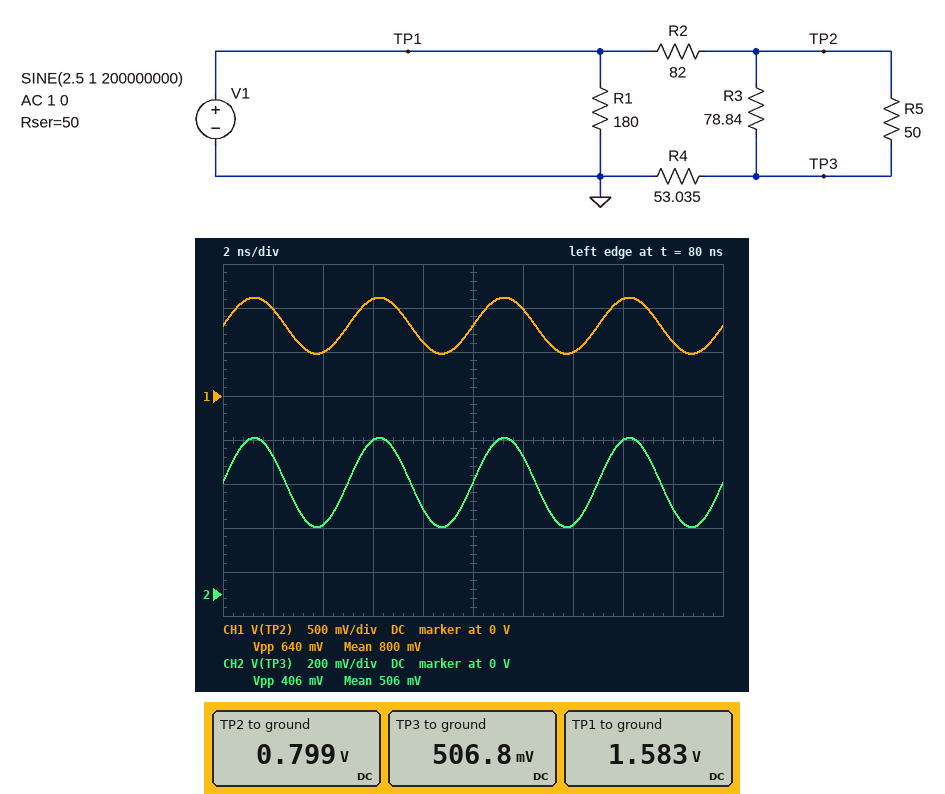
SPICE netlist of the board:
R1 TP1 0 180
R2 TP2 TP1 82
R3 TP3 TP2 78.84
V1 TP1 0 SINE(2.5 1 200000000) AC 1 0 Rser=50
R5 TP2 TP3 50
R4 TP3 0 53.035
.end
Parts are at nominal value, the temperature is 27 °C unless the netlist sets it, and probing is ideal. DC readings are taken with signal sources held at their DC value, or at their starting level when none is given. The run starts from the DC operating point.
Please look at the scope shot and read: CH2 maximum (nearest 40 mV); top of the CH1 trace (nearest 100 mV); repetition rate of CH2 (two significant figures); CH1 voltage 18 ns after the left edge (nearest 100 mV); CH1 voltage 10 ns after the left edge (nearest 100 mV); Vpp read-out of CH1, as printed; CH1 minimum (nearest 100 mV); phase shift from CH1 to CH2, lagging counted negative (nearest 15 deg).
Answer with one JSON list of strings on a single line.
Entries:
["720 mV", "1.1 V", "200 MHz", "600 mV", "800 mV", "640 mV", "500 mV", "0 deg"]
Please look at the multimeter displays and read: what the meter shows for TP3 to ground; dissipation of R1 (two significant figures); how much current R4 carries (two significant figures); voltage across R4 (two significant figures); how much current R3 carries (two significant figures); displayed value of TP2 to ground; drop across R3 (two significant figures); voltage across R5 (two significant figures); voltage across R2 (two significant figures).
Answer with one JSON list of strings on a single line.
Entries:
["506.8 mV", "14 mW", "9.6 mA", "510 mV", "3.7 mA", "0.799 V", "290 mV", "290 mV", "780 mV"]
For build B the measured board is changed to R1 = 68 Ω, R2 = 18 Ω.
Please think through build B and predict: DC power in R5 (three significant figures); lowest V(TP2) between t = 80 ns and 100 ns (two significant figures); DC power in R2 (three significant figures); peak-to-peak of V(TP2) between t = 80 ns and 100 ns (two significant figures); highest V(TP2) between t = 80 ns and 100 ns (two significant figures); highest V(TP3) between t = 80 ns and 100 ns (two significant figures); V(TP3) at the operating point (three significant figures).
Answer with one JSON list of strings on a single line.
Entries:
["2.28 mW", "550 mV", "2.20 mW", "740 mV", "1.3 V", "820 mV", "586 mV"]
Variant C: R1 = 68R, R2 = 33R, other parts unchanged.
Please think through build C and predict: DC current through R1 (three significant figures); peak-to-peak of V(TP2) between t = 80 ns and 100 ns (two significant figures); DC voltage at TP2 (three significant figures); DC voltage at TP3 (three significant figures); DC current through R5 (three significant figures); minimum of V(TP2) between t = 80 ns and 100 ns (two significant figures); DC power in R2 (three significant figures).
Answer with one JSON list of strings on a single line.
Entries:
["17.0 mA", "660 mV", "828 mV", "525 mV", "6.06 mA", "500 mV", "3.24 mW"]
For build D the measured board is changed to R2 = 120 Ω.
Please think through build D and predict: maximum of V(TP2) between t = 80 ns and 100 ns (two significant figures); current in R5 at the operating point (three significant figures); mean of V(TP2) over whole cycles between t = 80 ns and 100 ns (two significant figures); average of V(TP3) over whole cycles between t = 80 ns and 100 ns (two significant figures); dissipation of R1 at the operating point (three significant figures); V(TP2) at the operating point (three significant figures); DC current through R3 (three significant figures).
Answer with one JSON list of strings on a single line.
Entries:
["940 mV", "4.93 mA", "670 mV", "430 mV", "15.0 mW", "674 mV", "3.13 mA"]
